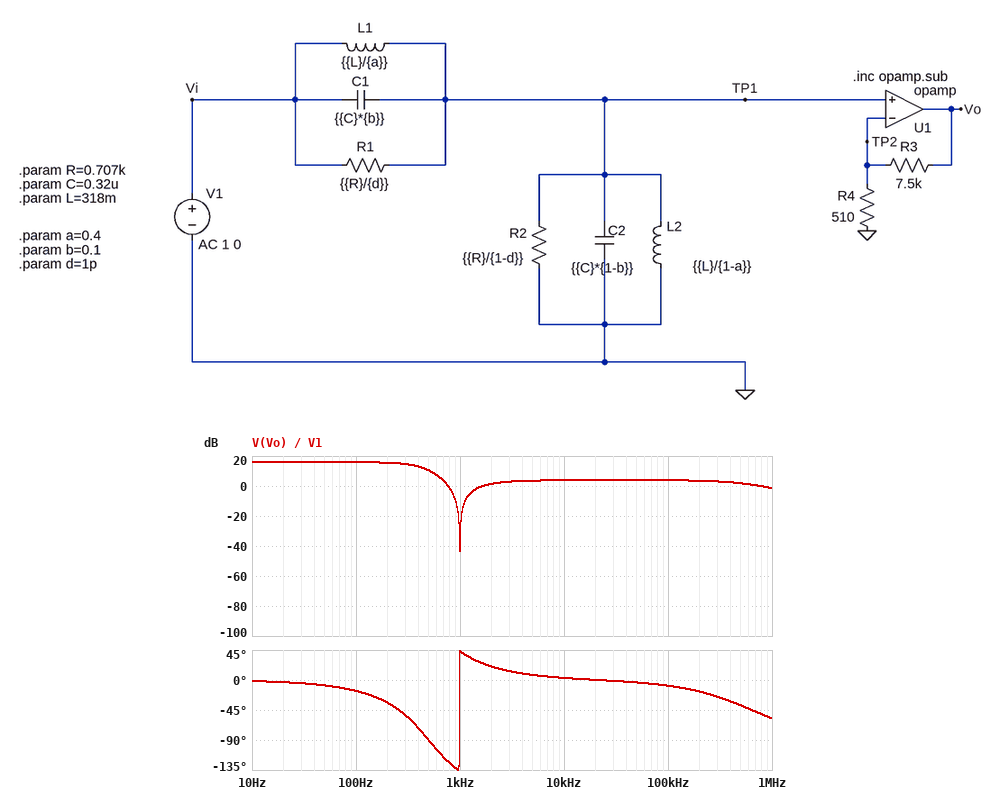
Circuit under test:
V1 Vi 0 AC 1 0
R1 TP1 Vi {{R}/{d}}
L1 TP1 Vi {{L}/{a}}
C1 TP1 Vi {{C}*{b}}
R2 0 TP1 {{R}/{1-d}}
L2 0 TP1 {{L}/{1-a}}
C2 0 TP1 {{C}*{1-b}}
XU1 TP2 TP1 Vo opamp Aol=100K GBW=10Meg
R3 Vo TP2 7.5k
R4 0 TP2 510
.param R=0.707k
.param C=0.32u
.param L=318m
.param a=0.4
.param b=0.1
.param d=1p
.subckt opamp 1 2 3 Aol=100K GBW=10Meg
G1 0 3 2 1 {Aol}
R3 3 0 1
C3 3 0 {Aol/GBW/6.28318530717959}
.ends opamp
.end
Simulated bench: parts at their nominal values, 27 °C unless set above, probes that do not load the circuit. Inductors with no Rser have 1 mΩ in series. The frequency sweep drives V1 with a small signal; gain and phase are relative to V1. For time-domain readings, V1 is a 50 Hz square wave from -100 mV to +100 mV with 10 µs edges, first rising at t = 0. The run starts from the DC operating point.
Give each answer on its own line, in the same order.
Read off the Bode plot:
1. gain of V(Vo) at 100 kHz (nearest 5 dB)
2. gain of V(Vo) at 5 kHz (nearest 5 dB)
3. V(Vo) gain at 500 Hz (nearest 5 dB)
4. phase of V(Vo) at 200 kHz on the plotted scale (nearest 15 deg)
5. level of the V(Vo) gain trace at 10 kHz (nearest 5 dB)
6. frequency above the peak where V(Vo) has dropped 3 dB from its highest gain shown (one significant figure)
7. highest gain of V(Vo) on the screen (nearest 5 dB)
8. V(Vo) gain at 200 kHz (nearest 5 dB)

5 dB
5 dB
10 dB
-15 deg
5 dB
400 Hz
15 dB
5 dB
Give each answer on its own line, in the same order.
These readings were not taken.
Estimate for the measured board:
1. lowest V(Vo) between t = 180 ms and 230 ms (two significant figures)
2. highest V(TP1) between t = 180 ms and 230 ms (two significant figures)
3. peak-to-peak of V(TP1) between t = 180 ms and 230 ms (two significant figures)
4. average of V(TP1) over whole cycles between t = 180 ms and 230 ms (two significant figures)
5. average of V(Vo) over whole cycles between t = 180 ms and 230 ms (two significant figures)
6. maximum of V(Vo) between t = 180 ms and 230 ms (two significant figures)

-830 mV
33 mV
86 mV
-10 mV
-160 mV
520 mV
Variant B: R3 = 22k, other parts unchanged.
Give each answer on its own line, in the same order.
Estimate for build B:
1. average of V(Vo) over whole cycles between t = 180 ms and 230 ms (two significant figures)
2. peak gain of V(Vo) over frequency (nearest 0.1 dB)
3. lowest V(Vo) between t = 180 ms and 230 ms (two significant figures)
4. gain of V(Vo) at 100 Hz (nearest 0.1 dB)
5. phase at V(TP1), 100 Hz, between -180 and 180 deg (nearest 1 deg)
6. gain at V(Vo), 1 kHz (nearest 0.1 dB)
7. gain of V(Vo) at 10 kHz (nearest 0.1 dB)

-440 mV
24.9 dB
-2.3 V
24.8 dB
-16 deg
-34.7 dB
12.8 dB
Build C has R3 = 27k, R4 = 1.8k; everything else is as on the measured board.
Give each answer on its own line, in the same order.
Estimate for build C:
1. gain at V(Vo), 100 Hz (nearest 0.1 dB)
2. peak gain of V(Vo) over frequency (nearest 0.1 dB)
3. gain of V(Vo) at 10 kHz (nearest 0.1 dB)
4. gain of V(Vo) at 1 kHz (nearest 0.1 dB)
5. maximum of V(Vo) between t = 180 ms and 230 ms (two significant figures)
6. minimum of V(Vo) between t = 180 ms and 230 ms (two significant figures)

16.0 dB
16.1 dB
4.0 dB
-43.5 dB
530 mV
-850 mV
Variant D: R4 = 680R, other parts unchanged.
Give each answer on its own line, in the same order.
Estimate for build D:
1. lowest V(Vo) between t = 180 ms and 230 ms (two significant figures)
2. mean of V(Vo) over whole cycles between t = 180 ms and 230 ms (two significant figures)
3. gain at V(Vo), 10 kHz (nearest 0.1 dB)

-640 mV
-120 mV
1.5 dB
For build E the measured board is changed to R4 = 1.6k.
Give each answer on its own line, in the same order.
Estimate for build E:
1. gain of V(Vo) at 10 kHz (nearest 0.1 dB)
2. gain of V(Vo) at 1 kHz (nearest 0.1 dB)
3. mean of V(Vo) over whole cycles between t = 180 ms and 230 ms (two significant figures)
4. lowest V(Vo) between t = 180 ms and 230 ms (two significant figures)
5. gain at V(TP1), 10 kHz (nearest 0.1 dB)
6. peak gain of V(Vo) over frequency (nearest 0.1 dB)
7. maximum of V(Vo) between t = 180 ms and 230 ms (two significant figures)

-5.0 dB
-52.5 dB
-57 mV
-300 mV
-20.1 dB
7.1 dB
190 mV
